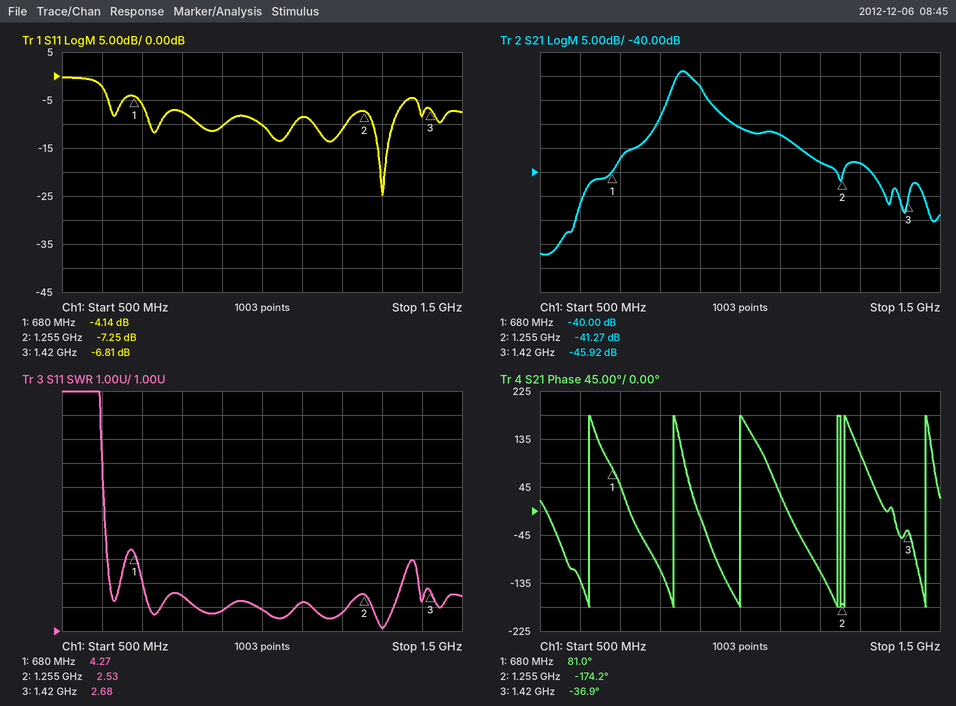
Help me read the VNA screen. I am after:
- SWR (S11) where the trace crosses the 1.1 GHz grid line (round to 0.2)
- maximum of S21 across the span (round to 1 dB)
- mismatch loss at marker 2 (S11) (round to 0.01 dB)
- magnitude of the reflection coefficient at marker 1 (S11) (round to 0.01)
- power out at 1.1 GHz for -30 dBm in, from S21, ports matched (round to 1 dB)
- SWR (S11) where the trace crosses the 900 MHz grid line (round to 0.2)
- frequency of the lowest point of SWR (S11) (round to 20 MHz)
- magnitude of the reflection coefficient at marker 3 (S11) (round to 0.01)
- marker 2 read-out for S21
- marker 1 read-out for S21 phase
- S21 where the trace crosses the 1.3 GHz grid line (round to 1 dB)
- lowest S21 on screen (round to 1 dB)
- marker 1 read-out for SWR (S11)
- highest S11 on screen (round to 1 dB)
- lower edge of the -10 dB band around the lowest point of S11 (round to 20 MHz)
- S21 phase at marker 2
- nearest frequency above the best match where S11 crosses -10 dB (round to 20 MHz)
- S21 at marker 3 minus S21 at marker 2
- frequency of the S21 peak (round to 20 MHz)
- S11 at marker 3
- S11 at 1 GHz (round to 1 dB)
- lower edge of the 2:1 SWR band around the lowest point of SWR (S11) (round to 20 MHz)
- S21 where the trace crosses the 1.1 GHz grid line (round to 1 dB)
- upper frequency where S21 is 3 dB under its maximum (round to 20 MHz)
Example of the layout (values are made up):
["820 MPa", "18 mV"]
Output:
["2.2", "-19 dB", "0.91 dB", "0.62", "-62 dBm", "1.8", "1.30 GHz", "0.46", "-41.27 dB", "81.0°", "-38 dB", "-57 dB", "4.27", "0 dB", "1.28 GHz", "-174.2°", "1.32 GHz", "-4.65 dB", "860 MHz", "-6.81 dB", "-10 dB", "1.28 GHz", "-32 dB", "900 MHz"]
